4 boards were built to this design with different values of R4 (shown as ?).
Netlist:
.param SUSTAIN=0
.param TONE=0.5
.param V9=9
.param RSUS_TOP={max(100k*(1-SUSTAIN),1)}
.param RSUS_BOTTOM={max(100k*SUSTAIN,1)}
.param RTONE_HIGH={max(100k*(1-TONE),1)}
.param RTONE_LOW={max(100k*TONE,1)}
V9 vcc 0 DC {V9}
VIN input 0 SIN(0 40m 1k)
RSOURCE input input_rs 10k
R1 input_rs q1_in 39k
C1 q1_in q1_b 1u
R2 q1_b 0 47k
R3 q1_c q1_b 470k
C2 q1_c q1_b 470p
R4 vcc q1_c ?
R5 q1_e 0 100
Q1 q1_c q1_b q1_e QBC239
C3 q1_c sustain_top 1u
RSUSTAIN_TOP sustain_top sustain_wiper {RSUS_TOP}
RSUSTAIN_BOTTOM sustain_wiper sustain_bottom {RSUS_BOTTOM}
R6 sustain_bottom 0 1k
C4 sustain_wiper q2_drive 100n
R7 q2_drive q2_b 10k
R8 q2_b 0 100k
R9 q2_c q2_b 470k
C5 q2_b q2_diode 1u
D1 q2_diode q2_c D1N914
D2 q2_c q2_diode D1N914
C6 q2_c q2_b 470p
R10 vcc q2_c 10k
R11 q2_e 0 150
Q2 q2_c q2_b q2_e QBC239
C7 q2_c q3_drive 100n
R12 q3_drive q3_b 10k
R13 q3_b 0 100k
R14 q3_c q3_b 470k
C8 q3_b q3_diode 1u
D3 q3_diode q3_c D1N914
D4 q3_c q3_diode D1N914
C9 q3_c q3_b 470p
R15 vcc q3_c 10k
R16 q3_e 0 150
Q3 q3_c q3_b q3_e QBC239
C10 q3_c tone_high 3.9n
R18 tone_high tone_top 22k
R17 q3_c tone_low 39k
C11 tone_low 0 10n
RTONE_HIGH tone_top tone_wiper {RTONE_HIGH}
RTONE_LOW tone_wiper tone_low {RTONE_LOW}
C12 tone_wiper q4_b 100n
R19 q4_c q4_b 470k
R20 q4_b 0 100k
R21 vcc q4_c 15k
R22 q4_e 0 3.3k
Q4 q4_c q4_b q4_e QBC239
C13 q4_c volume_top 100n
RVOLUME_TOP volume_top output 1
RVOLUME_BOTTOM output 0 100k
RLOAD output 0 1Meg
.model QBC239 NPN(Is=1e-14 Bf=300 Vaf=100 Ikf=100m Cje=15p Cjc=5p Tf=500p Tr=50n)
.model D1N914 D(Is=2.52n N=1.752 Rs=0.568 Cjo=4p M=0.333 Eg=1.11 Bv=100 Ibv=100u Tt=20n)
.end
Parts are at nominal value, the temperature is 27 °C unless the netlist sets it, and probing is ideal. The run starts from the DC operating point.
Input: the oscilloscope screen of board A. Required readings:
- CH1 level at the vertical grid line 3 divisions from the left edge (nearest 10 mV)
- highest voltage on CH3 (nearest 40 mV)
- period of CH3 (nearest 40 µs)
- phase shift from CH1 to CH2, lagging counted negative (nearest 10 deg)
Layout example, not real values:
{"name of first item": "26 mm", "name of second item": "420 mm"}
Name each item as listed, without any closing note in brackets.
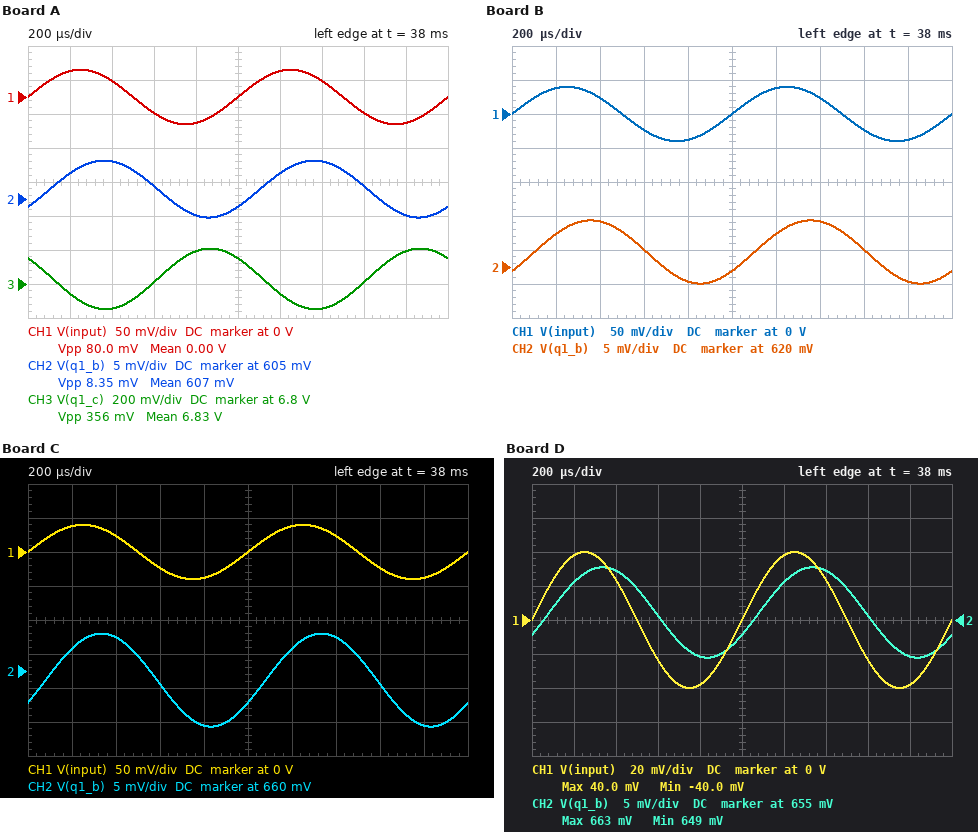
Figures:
{"CH1 level at the vertical grid line 3 divisions from the left edge": "-20 mV", "highest voltage on CH3": "7.00 V", "period of CH3": "1.00 ms", "phase shift from CH1 to CH2, lagging counted negative": "-40 deg"}
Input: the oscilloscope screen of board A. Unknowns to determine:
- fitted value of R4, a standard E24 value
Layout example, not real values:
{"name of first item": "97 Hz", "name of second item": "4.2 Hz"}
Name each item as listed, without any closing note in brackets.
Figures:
{"fitted value of R4, a standard E24 value": "18 kΩ"}
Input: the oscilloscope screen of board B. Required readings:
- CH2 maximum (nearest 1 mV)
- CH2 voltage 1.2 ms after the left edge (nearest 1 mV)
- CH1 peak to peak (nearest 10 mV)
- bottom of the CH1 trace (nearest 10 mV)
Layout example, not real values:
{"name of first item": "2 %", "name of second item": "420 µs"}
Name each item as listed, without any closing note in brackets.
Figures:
{"CH2 maximum": "627 mV", "CH2 voltage 1.2 ms after the left edge": "625 mV", "CH1 peak to peak": "80 mV", "bottom of the CH1 trace": "-40 mV"}
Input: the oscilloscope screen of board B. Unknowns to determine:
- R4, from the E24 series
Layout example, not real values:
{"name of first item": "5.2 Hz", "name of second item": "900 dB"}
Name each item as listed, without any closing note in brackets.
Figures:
{"R4, from the E24 series": "11 kΩ"}
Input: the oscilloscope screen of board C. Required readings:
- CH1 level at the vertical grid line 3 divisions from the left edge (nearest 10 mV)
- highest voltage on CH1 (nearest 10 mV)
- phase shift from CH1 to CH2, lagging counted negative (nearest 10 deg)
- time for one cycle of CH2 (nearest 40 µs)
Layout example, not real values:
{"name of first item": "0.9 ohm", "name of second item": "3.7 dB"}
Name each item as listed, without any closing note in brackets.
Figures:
{"CH1 level at the vertical grid line 3 divisions from the left edge": "-20 mV", "highest voltage on CH1": "40 mV", "phase shift from CH1 to CH2, lagging counted negative": "-30 deg", "time for one cycle of CH2": "1.00 ms"}
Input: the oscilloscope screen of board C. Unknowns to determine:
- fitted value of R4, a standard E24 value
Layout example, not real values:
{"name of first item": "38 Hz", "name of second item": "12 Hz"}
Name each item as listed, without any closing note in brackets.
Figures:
{"fitted value of R4, a standard E24 value": "3.6 kΩ"}
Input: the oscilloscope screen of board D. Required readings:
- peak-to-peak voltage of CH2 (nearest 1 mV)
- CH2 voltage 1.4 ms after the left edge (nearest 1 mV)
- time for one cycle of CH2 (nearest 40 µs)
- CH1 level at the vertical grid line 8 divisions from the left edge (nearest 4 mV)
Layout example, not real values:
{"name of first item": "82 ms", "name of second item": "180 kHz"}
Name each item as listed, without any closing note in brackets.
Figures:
{"peak-to-peak voltage of CH2": "13 mV", "CH2 voltage 1.4 ms after the left edge": "662 mV", "time for one cycle of CH2": "1.00 ms", "CH1 level at the vertical grid line 8 divisions from the left edge": "-24 mV"}
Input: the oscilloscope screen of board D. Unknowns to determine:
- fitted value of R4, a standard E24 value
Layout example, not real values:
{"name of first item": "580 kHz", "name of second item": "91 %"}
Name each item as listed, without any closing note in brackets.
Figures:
{"fitted value of R4, a standard E24 value": "3.9 kΩ"}
